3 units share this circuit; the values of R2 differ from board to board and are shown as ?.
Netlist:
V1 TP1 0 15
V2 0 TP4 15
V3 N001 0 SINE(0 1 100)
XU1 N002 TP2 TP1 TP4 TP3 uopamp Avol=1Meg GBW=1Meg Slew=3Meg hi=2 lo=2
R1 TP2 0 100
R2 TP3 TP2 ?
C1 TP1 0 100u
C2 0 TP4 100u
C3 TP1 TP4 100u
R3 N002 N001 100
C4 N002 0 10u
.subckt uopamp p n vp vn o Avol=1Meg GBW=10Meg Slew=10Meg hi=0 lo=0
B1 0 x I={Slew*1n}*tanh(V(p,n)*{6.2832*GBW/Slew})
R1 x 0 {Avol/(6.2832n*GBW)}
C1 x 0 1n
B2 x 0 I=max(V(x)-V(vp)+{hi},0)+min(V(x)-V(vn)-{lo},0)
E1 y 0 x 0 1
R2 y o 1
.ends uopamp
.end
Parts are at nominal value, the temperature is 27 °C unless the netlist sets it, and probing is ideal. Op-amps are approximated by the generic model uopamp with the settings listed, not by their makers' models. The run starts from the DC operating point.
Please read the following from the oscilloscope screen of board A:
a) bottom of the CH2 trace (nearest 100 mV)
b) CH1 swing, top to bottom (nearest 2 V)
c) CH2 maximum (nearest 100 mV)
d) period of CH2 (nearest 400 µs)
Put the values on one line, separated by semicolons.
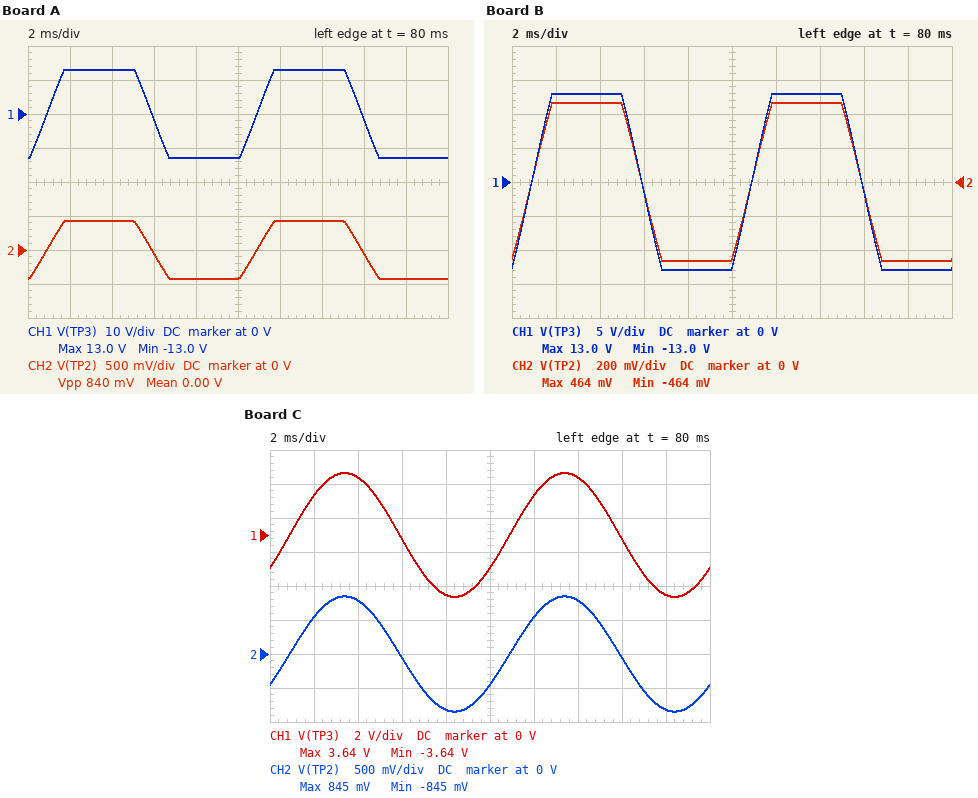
-400 mV; 26 V; 400 mV; 10.0 ms
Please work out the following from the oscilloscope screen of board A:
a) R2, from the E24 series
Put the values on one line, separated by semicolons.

3 kΩ
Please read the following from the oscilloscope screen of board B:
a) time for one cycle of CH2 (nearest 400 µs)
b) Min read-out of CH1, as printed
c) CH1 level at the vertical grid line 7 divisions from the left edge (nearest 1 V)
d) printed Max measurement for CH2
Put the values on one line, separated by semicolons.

10.0 ms; -13.0 V; 13 V; 464 mV
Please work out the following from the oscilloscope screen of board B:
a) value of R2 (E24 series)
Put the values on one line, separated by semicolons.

2.7 kΩ
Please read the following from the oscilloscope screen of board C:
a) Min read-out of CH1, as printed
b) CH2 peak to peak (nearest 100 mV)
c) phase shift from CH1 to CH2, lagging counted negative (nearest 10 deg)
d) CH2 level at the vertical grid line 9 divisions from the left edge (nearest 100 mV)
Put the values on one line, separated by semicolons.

-3.64 V; 1.7 V; 0 deg; -800 mV
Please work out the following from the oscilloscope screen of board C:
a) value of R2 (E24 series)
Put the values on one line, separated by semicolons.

330 Ω
